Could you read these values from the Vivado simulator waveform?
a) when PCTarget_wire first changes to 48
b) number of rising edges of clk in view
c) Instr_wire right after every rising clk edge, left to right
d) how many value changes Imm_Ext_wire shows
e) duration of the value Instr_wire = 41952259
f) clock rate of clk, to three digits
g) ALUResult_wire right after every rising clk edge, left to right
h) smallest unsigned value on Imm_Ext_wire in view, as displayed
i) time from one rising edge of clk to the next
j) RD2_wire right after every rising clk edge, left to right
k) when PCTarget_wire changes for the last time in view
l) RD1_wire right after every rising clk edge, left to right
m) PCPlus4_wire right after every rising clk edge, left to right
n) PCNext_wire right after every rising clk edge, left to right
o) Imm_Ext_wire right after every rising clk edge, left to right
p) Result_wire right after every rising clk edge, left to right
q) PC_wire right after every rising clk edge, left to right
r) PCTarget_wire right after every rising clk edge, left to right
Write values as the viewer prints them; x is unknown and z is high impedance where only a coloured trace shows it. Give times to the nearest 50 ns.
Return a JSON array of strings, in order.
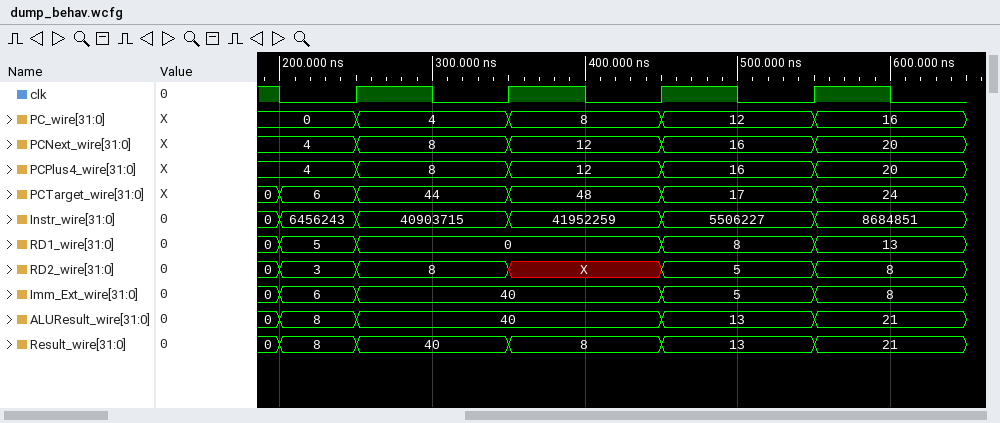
["350 ns", "4", "40903715, 41952259, 5506227, 8684851", "4", "100 ns", "10.0 MHz", "40, 40, 13, 21", "0", "100 ns", "8, X, 5, 8", "550 ns", "0, 0, 8, 13", "8, 12, 16, 20", "8, 12, 16, 20", "40, 40, 5, 8", "40, 8, 13, 21", "4, 8, 12, 16", "44, 48, 17, 24"]
